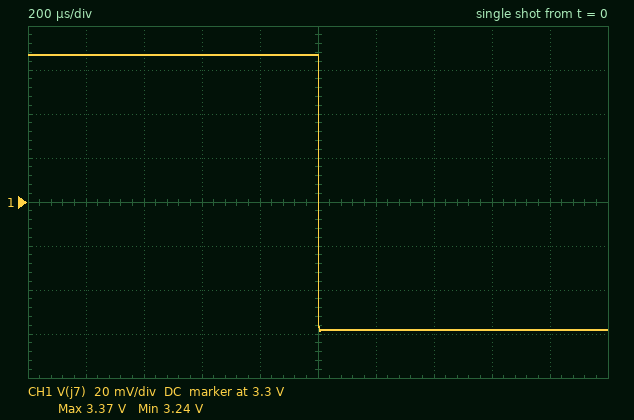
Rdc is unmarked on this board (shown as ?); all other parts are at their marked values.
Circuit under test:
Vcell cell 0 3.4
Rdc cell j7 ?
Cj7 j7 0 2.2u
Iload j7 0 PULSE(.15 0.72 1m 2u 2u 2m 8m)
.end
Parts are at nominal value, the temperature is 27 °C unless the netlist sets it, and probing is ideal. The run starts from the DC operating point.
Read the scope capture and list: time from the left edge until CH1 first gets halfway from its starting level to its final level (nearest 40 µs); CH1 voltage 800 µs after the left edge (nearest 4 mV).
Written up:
1.00 ms
3.368 V
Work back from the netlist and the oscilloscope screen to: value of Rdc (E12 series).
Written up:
0.22 Ω
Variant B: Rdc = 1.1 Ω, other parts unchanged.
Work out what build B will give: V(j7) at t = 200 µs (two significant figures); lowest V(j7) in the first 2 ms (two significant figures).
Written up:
3.2 V
2.6 V
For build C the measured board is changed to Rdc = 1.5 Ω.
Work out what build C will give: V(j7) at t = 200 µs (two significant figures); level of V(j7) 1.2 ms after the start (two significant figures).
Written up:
3.2 V
2.3 V
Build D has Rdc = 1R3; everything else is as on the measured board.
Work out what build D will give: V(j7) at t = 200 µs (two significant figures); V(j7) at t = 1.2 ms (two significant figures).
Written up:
3.2 V
2.5 V
